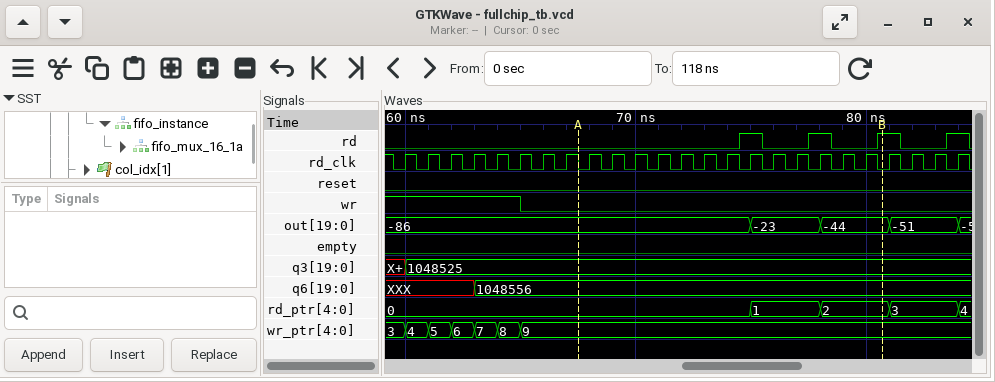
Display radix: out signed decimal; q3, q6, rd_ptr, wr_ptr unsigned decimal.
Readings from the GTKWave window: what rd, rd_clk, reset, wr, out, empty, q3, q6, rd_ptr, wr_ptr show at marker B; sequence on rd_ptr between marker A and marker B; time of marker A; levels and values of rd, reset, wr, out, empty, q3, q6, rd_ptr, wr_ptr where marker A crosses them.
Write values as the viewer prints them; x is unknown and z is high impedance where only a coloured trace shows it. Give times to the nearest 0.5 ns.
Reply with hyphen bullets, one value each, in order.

- rd=1, rd_clk=0, reset=0, wr=0, out=-44, empty=0, q3=1048525, q6=1048556, rd_ptr=2, wr_ptr=9
- 0, 1, 2
- 67.5 ns
- rd=0, reset=0, wr=0, out=-86, empty=0, q3=1048525, q6=1048556, rd_ptr=0, wr_ptr=9
